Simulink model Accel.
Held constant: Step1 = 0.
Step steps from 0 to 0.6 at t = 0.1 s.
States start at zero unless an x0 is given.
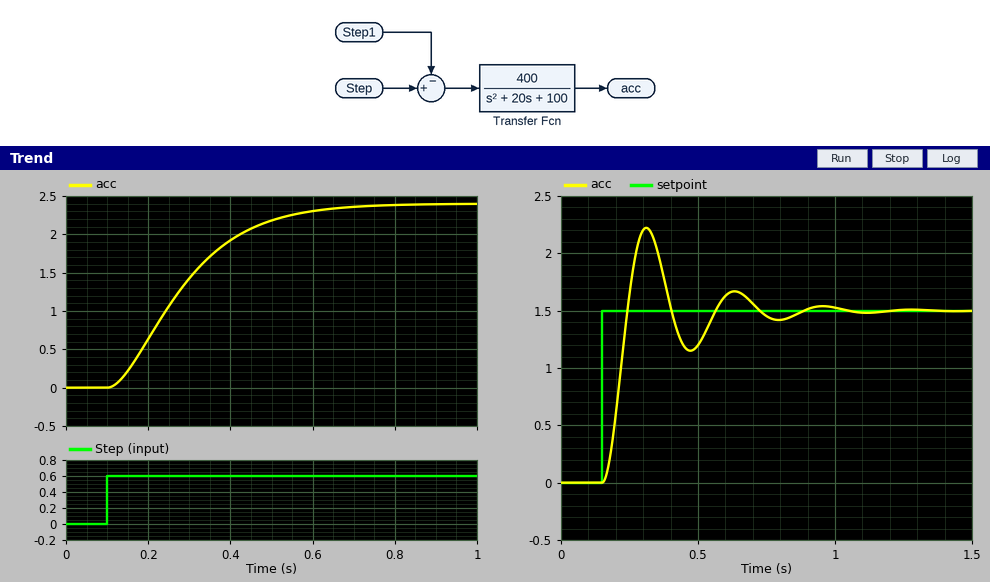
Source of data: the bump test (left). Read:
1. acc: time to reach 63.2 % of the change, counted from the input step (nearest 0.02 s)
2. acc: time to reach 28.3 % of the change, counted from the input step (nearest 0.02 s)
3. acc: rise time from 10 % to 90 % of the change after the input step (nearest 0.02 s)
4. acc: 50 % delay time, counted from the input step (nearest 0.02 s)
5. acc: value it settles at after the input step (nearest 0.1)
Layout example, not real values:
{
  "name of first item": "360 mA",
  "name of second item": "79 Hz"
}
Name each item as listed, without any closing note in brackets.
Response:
{
  "acc: time to reach 63.2 % of the change, counted from the input step": "0.22 s",
  "acc: time to reach 28.3 % of the change, counted from the input step": "0.10 s",
  "acc: rise time from 10 % to 90 % of the change after the input step": "0.34 s",
  "acc: 50 % delay time, counted from the input step": "0.16 s",
  "acc: value it settles at after the input step": "2.4"
}
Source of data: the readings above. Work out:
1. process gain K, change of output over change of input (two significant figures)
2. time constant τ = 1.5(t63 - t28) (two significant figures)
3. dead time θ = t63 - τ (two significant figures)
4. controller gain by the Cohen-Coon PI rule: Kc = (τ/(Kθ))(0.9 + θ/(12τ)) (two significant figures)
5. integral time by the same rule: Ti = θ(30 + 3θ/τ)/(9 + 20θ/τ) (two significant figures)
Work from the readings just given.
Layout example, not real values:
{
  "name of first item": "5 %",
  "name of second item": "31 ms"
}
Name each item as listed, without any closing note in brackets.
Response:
{
  "process gain K, change of output over change of input": "4.0",
  "time constant τ = 1.5(t63 - t28)": "0.18 s",
  "dead time θ = t63 - τ": "0.040 s",
  "controller gain by the Cohen-Coon PI rule: Kc = (τ/(Kθ))(0.9 + θ/(12τ))": "1.0",
  "integral time by the same rule: Ti = θ(30 + 3θ/τ)/(9 + 20θ/τ)": "0.091 s"
}
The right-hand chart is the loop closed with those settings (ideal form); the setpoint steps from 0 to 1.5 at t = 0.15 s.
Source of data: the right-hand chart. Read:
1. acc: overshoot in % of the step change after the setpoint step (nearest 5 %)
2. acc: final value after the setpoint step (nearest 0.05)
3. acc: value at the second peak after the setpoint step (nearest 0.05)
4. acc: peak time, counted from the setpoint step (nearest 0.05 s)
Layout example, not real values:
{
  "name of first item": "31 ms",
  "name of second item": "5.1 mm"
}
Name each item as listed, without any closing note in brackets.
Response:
{
  "acc: overshoot in % of the step change after the setpoint step": "50 %",
  "acc: final value after the setpoint step": "1.50",
  "acc: value at the second peak after the setpoint step": "1.65",
  "acc: peak time, counted from the setpoint step": "0.15 s"
}
